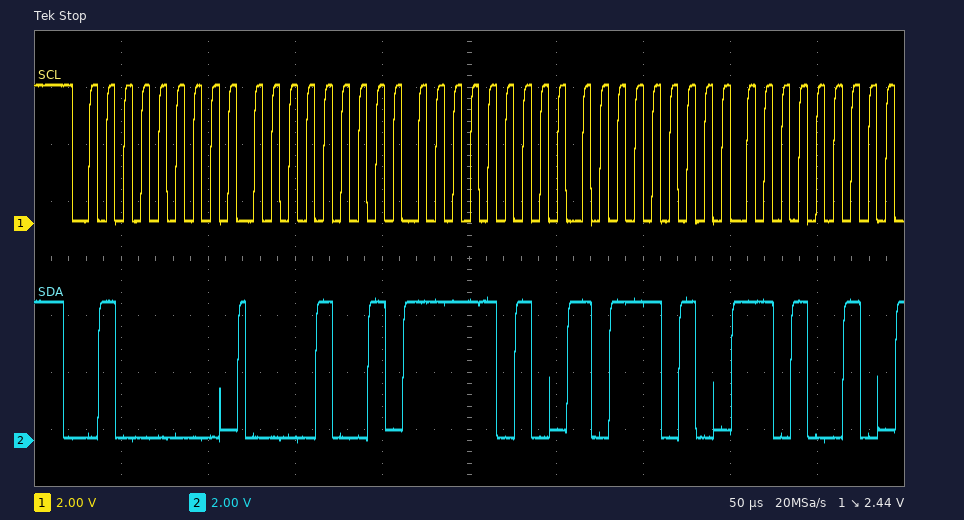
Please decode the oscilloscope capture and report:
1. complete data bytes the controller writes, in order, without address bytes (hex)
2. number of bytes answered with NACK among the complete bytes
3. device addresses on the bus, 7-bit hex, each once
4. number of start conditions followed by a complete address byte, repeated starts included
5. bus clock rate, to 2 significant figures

09 FA BA D2
0
0x20
1
100 kHz
